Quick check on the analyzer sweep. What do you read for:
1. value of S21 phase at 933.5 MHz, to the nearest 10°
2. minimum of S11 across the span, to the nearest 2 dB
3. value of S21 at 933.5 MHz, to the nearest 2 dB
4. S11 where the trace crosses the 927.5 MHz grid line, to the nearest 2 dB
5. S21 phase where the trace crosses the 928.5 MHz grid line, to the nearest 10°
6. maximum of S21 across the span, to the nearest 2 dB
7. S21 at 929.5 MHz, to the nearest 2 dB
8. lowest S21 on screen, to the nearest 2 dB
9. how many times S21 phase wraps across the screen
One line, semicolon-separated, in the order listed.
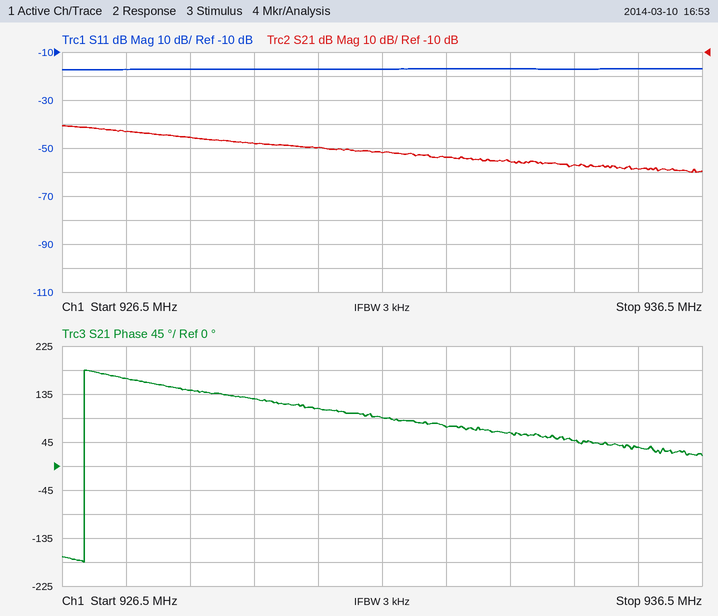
60°; -18 dB; -56 dB; -18 dB; 140°; -40 dB; -48 dB; -60 dB; 1
